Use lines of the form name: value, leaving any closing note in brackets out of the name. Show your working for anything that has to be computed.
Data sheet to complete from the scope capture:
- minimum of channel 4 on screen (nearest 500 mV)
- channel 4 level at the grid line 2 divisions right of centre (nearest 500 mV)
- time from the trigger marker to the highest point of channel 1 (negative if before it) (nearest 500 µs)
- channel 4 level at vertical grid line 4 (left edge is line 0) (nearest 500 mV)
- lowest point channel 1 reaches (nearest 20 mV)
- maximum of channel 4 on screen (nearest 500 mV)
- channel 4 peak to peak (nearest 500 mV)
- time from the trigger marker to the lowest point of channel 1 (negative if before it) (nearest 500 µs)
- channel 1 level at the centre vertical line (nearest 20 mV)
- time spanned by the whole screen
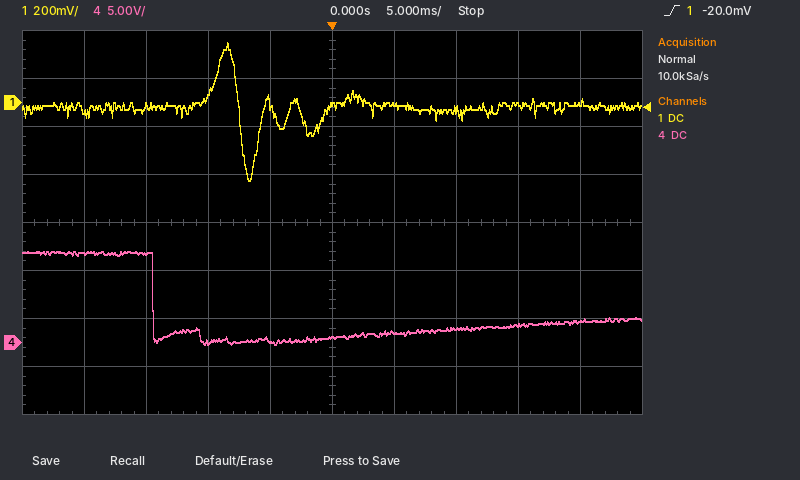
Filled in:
minimum of channel 4 on screen: 0.0 V
channel 4 level at the grid line 2 divisions right of centre: 1.5 V
time from the trigger marker to the highest point of channel 1 (negative if before it): -8.5 ms
channel 4 level at vertical grid line 4 (left edge is line 0): 0.0 V
lowest point channel 1 reaches: -320 mV
maximum of channel 4 on screen: 9.5 V
channel 4 peak to peak: 9.5 V − (0.0 V) = 9.5 V
time from the trigger marker to the lowest point of channel 1 (negative if before it): -6.5 ms
channel 1 level at the centre vertical line: -20 mV
time spanned by the whole screen: 50 ms
